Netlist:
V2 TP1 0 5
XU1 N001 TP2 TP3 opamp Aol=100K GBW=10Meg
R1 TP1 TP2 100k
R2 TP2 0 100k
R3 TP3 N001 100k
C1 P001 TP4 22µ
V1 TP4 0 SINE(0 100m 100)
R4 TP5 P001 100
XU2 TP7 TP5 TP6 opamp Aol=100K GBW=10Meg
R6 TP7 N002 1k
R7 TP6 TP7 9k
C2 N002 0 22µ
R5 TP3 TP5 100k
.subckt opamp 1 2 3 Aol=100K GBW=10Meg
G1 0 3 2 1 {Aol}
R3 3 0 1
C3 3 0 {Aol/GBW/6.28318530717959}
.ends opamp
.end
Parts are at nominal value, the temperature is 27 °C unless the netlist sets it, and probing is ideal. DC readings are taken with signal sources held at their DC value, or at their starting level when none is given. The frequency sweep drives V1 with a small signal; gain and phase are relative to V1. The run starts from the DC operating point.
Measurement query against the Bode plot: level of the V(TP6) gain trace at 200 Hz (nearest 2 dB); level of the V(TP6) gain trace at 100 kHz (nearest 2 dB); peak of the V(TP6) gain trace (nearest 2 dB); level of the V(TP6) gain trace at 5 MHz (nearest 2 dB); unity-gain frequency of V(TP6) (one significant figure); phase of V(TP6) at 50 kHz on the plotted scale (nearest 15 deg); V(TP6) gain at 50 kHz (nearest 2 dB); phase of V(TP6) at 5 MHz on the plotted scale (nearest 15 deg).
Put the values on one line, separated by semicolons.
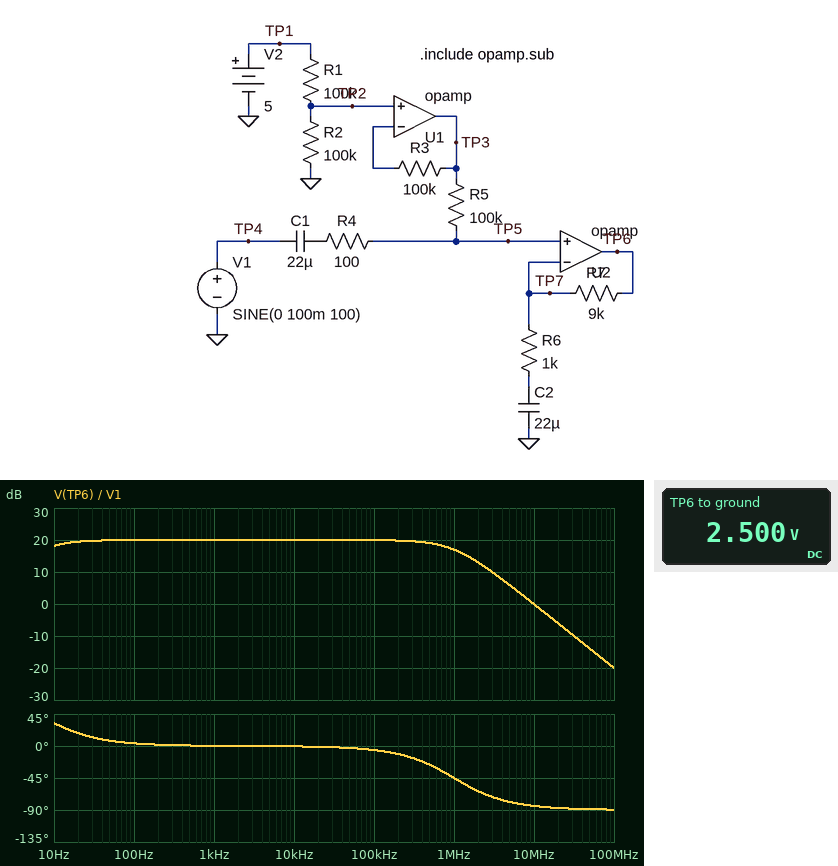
20 dB; 20 dB; 20 dB; 6 dB; 10 MHz; 0 deg; 20 dB; -75 deg
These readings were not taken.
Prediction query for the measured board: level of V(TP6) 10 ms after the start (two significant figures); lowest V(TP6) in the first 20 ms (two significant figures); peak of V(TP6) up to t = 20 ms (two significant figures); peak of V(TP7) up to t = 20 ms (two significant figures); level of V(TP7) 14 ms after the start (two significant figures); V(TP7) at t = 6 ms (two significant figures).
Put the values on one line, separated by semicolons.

2.5 V; 1.5 V; 3.5 V; 2.6 V; 2.6 V; 2.4 V
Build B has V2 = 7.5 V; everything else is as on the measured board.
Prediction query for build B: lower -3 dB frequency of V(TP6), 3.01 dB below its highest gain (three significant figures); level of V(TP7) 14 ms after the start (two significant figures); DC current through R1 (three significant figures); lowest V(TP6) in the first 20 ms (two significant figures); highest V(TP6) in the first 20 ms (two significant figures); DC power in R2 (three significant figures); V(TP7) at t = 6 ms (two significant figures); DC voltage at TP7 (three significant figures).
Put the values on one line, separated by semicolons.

7.16 Hz; 3.8 V; 37.5 µA; 2.7 V; 4.7 V; 141 µW; 3.7 V; 3.75 V
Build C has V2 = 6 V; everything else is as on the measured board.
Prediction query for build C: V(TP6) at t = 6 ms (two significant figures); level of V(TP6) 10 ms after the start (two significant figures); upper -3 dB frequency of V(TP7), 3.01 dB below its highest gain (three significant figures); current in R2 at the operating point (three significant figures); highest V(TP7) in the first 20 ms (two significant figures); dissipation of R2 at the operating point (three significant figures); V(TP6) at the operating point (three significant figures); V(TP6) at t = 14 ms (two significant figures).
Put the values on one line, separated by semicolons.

2.3 V; 3.0 V; 1.00 MHz; 30.0 µA; 3.1 V; 90.0 µW; 3.00 V; 3.5 V
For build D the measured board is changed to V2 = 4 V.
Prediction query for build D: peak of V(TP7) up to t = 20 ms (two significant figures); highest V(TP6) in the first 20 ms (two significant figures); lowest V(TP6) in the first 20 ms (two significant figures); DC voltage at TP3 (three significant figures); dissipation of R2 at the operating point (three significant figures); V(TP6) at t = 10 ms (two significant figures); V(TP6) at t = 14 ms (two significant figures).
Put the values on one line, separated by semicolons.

2.1 V; 3.0 V; 960 mV; 2.00 V; 40.0 µW; 2.0 V; 2.5 V
